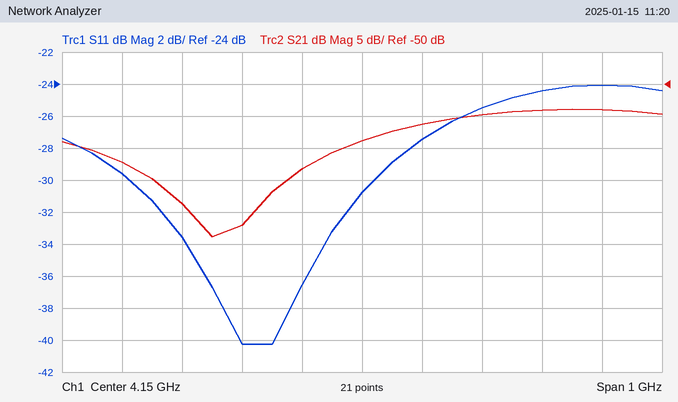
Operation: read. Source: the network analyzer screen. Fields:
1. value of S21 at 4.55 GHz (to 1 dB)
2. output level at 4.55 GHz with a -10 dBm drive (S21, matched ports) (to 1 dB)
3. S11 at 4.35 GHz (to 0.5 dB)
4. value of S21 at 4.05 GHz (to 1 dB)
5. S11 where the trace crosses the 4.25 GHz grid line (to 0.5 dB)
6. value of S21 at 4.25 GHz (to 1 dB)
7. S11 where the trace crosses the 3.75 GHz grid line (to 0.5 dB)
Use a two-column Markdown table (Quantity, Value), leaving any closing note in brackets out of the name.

| Quantity | Value |
|---|---|
| value of S21 at 4.55 GHz | -54 dB |
| output level at 4.55 GHz with a -10 dBm drive (S21, matched ports) | -64 dBm |
| S11 at 4.35 GHz | -25.5 dB |
| value of S21 at 4.05 GHz | -63 dB |
| S11 where the trace crosses the 4.25 GHz grid line | -27.5 dB |
| value of S21 at 4.25 GHz | -56 dB |
| S11 where the trace crosses the 3.75 GHz grid line | -29.5 dB |
